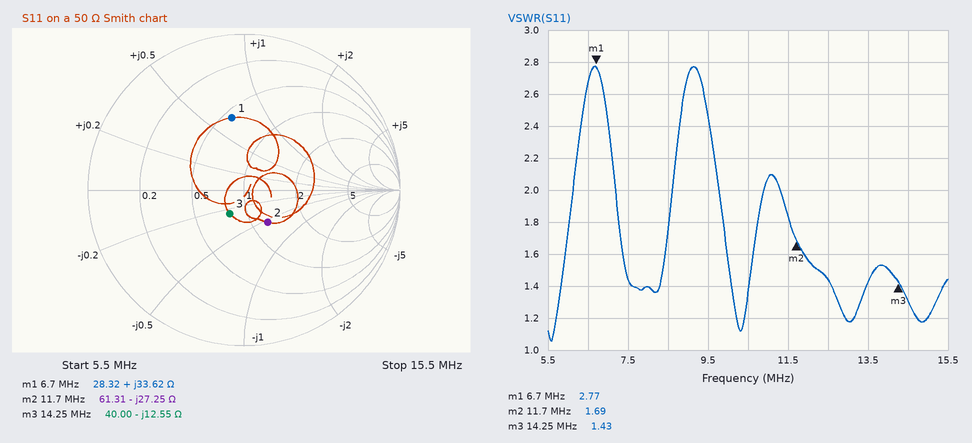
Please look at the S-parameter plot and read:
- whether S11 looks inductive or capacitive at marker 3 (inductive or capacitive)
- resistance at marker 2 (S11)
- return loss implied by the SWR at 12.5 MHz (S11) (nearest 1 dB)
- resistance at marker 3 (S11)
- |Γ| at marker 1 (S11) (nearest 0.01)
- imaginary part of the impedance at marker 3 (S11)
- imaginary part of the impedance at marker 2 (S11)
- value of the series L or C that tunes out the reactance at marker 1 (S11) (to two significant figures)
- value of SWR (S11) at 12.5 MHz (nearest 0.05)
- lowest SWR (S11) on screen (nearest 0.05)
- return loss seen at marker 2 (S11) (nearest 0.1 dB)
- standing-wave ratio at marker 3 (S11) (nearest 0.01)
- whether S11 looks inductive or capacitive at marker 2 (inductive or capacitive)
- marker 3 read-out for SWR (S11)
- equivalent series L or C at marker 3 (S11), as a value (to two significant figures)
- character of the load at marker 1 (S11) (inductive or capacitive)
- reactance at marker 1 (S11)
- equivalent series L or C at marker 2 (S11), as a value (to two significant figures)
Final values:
capacitive
61.31 Ω
15 dB
40.00 Ω
0.47
-12.55 Ω
-27.25 Ω
710 pF
1.45
1.05
11.8 dB
1.43
capacitive
1.43
890 pF
inductive
+33.62 Ω
500 pF
